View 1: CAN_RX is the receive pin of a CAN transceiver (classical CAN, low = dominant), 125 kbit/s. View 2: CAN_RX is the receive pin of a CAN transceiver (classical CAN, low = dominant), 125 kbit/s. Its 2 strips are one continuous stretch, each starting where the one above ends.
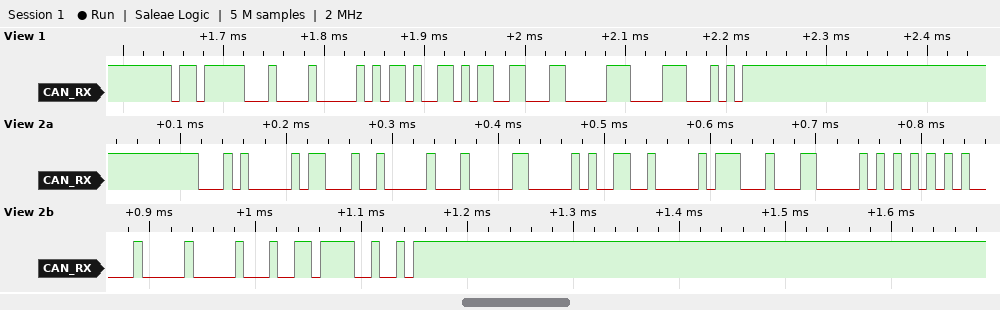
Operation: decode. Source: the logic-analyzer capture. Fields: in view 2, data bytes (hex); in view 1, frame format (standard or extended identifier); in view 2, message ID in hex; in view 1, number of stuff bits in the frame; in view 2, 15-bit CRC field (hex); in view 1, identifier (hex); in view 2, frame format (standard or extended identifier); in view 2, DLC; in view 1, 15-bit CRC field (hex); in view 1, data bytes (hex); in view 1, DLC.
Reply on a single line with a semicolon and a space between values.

13 20 71 18 15 54 00 00; standard; 0x05004804; 3; 0x4DE4; 0x6F9; extended; 8; 0x30E2; 0B 4D 66 30; 4
